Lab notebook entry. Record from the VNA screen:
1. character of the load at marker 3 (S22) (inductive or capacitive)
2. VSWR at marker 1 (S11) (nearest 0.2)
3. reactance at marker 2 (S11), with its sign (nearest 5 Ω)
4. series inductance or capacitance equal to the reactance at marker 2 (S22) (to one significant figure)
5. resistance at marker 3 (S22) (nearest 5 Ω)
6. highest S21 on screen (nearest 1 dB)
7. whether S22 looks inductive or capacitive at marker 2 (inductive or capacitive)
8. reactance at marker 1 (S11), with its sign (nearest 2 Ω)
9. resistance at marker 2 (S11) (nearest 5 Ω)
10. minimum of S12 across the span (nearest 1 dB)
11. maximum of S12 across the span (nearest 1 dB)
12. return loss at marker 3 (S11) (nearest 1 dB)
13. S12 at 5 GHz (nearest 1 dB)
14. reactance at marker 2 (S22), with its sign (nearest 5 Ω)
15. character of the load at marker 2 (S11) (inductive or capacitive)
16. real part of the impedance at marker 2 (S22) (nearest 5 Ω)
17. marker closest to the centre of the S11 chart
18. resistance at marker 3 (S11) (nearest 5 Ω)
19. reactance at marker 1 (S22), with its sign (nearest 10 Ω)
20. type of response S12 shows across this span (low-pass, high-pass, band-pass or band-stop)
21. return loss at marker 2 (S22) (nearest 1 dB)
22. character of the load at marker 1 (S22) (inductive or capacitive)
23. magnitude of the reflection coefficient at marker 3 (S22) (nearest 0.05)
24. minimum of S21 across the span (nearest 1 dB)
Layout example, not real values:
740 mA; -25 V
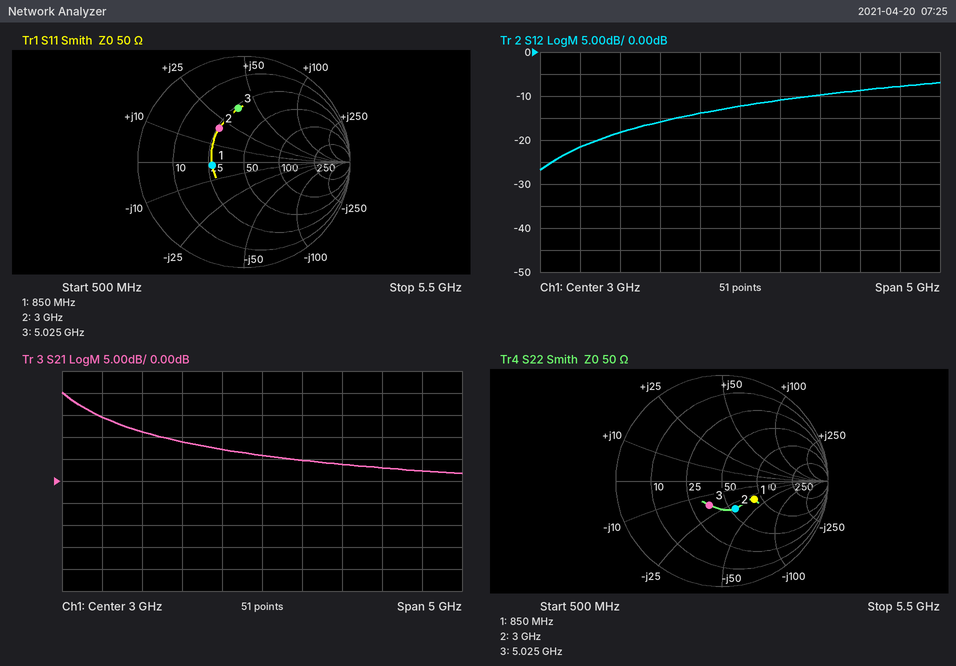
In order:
capacitive; 1.8; +20 Ω; 2 pF; 35 Ω; 20 dB; capacitive; -2 Ω; 25 Ω; -27 dB; -7 dB; 6 dB; -8 dB; -30 Ω; inductive; 55 Ω; marker 1; 25 Ω; -30 Ω; high-pass; 11 dB; capacitive; 0.25; 2 dB
